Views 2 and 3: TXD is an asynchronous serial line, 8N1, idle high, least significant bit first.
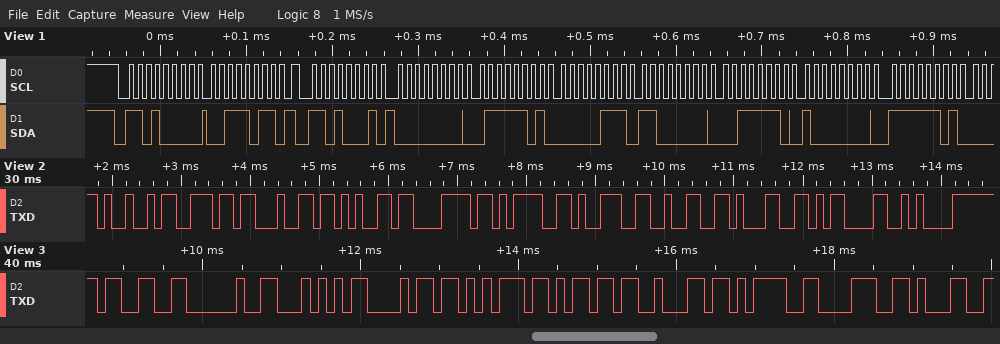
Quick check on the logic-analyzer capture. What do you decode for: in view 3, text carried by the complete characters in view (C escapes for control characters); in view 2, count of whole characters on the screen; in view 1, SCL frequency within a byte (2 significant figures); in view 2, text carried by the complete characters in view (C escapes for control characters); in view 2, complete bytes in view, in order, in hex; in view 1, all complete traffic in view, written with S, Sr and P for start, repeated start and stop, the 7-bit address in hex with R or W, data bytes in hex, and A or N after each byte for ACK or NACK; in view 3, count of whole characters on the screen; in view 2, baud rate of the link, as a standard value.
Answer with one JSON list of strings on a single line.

["\"3 Thumb=81\"", "11", "100 kHz", "\"Index=921\\r\\n\"", "49 6E 64 65 78 3D 39 32 31 0D 0A", "S 68W A 3B A Sr 68R A 00 A 7D A 07 A C0 A 3E A 80 A FD A", "10", "9600 baud"]
